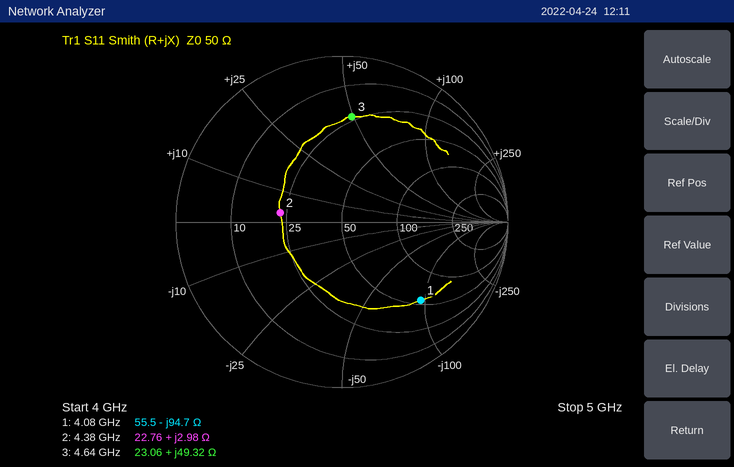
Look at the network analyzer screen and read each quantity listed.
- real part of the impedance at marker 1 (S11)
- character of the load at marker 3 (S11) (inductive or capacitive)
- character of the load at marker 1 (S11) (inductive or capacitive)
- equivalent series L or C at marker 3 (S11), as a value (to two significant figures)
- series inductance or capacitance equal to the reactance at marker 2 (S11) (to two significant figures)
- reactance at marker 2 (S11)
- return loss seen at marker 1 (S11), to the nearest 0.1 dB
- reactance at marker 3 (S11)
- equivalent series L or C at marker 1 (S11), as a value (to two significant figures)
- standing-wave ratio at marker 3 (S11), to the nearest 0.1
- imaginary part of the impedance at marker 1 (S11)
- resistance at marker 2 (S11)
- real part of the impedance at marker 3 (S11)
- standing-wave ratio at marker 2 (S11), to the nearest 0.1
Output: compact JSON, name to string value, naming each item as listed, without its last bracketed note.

{"real part of the impedance at marker 1": "55.5 Ω", "character of the load at marker 3 (S11)": "inductive", "character of the load at marker 1 (S11)": "capacitive", "equivalent series L or C at marker 3 (S11), as a value": "1.7 nH", "series inductance or capacitance equal to the reactance at marker 2 (S11)": "110 pH", "reactance at marker 2": "+2.98 Ω", "return loss seen at marker 1 (S11), to the nearest 0.1 dB": "3.5 dB", "reactance at marker 3": "+49.32 Ω", "equivalent series L or C at marker 1 (S11), as a value": "410 fF", "standing-wave ratio at marker 3 (S11), to the nearest 0.1": "4.5", "imaginary part of the impedance at marker 1": "-94.7 Ω", "resistance at marker 2": "22.76 Ω", "real part of the impedance at marker 3": "23.06 Ω", "standing-wave ratio at marker 2 (S11), to the nearest 0.1": "2.2"}
